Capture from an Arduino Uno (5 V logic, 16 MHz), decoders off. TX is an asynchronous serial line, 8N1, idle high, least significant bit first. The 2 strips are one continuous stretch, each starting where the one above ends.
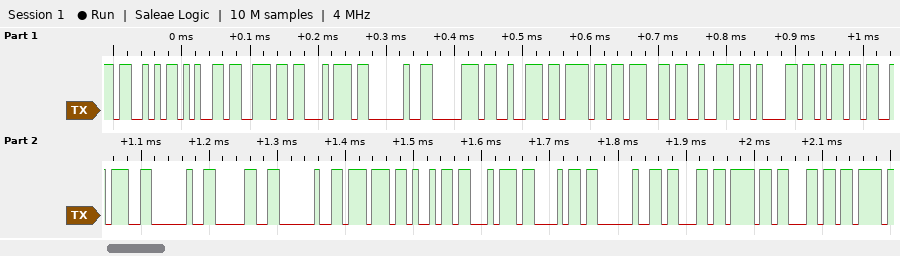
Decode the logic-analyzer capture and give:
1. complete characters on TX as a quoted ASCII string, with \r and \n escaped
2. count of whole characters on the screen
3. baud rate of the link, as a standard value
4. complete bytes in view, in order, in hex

"Sent program: 0 with col"
24
115200 baud
53 65 6E 74 20 70 72 6F 67 72 61 6D 3A 20 30 20 77 69 74 68 20 63 6F 6C
